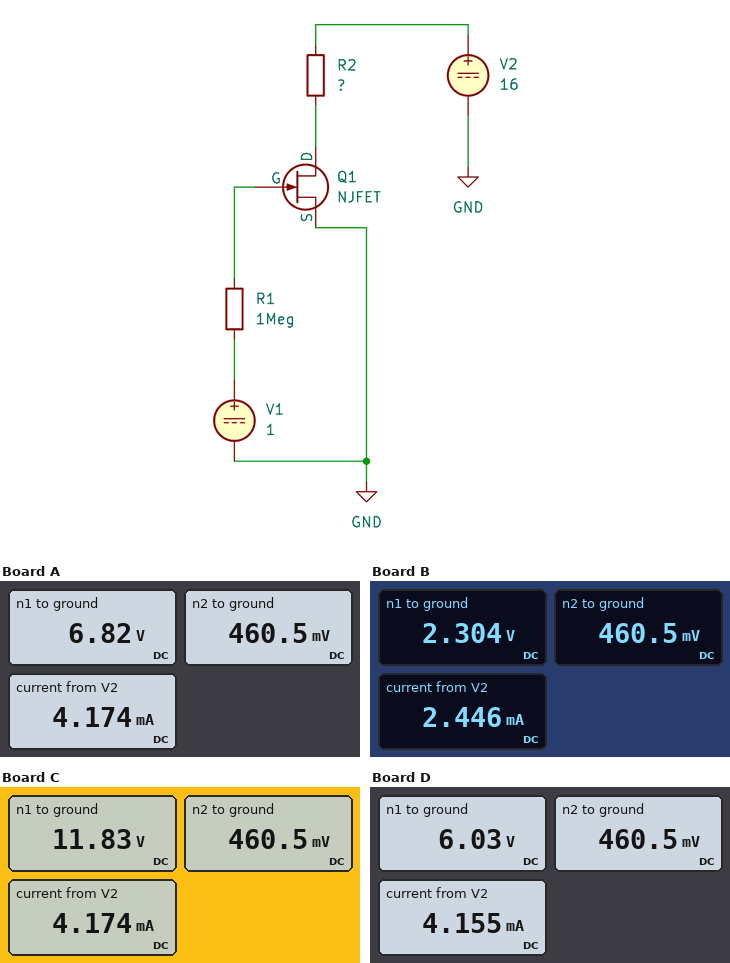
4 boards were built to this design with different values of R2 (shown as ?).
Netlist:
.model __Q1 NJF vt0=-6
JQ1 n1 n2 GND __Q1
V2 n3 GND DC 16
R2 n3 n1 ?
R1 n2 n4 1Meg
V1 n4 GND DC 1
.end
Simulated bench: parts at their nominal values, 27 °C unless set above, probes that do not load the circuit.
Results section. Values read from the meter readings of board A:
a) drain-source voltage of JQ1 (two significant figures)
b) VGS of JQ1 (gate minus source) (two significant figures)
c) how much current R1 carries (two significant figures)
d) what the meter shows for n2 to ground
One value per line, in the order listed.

6.8 V
460 mV
540 nA
460.5 mV
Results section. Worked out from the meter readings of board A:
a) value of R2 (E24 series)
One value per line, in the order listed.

2.2 kΩ
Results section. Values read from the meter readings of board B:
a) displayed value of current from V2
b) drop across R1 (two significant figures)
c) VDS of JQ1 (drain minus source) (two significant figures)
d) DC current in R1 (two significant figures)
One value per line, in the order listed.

2.446 mA
540 mV
2.3 V
540 nA
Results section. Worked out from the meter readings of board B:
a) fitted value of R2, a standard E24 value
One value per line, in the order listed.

5.6 kΩ
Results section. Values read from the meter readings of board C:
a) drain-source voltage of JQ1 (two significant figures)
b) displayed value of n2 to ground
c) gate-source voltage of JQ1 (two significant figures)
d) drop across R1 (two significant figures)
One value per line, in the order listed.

12 V
460.5 mV
460 mV
540 mV
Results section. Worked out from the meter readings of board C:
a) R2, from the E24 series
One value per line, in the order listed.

1 kΩ
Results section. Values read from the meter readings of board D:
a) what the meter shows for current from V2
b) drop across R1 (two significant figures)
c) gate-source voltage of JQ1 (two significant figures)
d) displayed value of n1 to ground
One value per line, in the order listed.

4.155 mA
540 mV
460 mV
6.03 V
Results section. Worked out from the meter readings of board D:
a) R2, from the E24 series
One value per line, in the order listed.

2.4 kΩ
